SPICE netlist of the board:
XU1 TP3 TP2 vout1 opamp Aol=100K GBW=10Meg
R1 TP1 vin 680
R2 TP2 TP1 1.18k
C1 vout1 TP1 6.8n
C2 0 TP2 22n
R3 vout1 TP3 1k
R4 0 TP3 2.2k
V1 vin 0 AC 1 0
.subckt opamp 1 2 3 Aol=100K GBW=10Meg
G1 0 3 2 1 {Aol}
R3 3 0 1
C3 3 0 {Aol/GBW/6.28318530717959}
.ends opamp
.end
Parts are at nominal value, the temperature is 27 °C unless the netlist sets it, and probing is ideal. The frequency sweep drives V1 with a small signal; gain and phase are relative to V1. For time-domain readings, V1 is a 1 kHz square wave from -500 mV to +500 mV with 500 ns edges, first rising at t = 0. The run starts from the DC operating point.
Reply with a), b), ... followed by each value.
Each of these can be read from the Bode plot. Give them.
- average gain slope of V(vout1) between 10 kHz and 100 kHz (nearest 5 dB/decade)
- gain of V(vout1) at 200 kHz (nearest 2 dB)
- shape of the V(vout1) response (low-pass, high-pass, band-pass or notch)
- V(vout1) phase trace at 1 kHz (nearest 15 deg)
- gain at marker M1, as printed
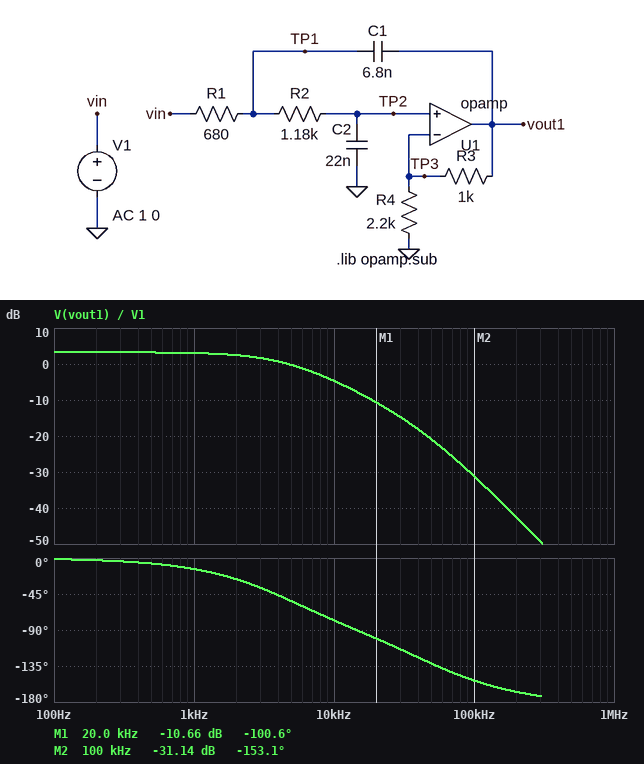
a) -25 dB/decade
b) -42 dB
c) low-pass
d) -15 deg
e) -10.66 dB
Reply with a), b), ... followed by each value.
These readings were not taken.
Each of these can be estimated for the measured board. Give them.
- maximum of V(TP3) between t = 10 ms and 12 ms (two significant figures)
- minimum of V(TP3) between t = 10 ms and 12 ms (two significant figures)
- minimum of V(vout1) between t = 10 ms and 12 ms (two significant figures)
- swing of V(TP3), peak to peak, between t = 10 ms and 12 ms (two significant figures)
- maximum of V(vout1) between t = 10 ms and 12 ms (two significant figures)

a) 500 mV
b) -500 mV
c) -730 mV
d) 1.0 V
e) 730 mV
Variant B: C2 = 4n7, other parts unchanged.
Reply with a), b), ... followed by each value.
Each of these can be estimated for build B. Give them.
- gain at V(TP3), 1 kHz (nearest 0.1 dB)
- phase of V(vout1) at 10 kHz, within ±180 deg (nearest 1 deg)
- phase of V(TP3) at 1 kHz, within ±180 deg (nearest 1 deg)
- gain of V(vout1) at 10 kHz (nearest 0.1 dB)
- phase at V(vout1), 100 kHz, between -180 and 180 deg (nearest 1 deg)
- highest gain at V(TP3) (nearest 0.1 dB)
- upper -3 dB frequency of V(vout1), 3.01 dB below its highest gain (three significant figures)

a) 0 dB
b) -25 deg
c) -2 deg
d) 3.3 dB
e) -156 deg
f) 0.1 dB
g) 33.4 kHz
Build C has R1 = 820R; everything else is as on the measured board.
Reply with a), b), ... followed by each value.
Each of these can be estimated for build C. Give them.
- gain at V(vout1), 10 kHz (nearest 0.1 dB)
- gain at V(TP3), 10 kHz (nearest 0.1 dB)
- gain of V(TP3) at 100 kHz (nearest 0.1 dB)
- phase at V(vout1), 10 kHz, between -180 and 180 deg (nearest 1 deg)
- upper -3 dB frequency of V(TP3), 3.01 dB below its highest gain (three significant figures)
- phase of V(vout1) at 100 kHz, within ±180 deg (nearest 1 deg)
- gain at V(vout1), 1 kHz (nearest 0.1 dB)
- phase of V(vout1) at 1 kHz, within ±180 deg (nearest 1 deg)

a) -5.2 dB
b) -8.4 dB
c) -35.8 dB
d) -81 deg
e) 4.19 kHz
f) -156 deg
g) 3.0 dB
h) -15 deg
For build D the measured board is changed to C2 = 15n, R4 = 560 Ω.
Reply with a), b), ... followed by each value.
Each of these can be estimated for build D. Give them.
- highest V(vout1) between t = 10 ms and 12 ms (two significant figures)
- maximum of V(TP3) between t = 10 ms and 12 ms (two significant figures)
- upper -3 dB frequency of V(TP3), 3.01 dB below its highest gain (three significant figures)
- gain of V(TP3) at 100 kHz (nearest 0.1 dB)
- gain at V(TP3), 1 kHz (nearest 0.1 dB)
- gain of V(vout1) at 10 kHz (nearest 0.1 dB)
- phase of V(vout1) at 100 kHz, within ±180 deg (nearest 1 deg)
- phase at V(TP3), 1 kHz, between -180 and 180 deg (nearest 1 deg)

a) 1.4 V
b) 500 mV
c) 10.1 kHz
d) -30.6 dB
e) 0 dB
f) 5.9 dB
g) -160 deg
h) -7 deg
